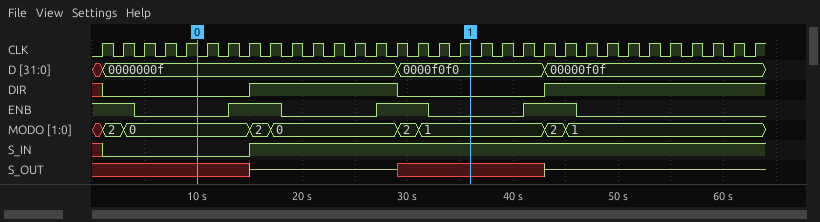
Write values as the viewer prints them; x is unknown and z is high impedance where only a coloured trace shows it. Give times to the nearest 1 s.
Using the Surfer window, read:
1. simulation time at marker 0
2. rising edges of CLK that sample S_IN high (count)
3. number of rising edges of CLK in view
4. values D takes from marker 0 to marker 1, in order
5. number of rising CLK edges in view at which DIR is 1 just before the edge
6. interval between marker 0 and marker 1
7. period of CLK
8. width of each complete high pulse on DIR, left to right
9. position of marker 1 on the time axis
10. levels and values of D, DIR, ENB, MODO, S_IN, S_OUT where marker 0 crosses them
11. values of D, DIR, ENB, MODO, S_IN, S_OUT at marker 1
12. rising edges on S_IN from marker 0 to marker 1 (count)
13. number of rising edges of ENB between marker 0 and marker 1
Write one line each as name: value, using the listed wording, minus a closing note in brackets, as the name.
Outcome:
simulation time at marker 0: 10 s
rising edges of CLK that sample S_IN high: 24
number of rising edges of CLK in view: 32
values D takes from marker 0 to marker 1, in order: 0000000f, 0000f0f0
number of rising CLK edges in view at which DIR is 1 just before the edge: 17
interval between marker 0 and marker 1: 26 s
period of CLK: 2 s
width of each complete high pulse on DIR, left to right: 14 s
position of marker 1 on the time axis: 36 s
levels and values of D, DIR, ENB, MODO, S_IN, S_OUT where marker 0 crosses them: D=0000000f, DIR=0, ENB=0, MODO=0, S_IN=0, S_OUT=x
values of D, DIR, ENB, MODO, S_IN, S_OUT at marker 1: D=0000f0f0, DIR=0, ENB=0, MODO=1, S_IN=1, S_OUT=x
rising edges on S_IN from marker 0 to marker 1: 1
number of rising edges of ENB between marker 0 and marker 1: 2
